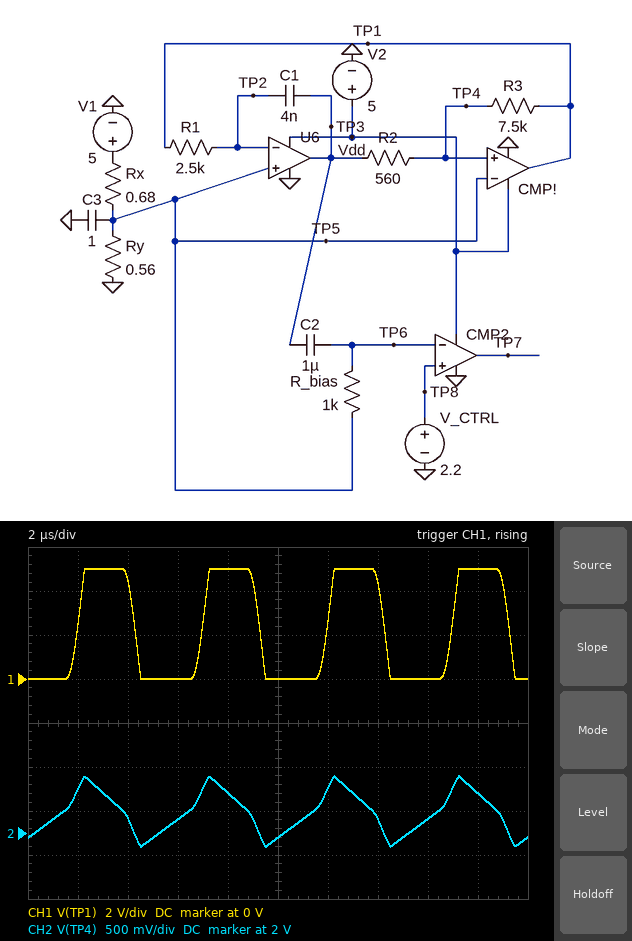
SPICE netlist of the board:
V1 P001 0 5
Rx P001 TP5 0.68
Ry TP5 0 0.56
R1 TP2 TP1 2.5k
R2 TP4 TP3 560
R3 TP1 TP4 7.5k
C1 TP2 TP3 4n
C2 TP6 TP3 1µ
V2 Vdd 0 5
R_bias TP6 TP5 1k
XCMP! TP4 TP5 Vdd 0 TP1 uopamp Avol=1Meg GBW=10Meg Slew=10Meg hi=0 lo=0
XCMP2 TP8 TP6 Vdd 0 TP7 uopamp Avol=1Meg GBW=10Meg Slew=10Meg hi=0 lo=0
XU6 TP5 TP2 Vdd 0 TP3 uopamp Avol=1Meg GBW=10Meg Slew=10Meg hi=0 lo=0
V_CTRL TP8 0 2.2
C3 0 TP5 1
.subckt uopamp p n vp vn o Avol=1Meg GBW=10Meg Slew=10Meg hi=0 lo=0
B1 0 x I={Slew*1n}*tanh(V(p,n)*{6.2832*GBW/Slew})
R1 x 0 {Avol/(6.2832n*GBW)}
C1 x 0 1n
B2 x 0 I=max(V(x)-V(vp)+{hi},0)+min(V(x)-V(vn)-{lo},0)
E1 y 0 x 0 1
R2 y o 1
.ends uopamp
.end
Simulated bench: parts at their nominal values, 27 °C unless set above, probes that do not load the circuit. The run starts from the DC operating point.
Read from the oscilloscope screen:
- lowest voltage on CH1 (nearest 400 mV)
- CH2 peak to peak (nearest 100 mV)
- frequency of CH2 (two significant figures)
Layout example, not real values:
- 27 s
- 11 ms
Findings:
- 0 V
- 800 mV
- 200 kHz
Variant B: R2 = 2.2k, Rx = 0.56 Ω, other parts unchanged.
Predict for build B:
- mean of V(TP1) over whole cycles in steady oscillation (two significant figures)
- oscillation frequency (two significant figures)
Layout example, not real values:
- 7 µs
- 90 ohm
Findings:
- 2.5 V
- 75 kHz
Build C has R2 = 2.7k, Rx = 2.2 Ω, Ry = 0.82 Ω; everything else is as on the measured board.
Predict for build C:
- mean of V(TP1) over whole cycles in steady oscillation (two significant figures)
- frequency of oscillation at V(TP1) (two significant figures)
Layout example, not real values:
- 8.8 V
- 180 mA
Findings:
- 1.4 V
- 50 kHz
